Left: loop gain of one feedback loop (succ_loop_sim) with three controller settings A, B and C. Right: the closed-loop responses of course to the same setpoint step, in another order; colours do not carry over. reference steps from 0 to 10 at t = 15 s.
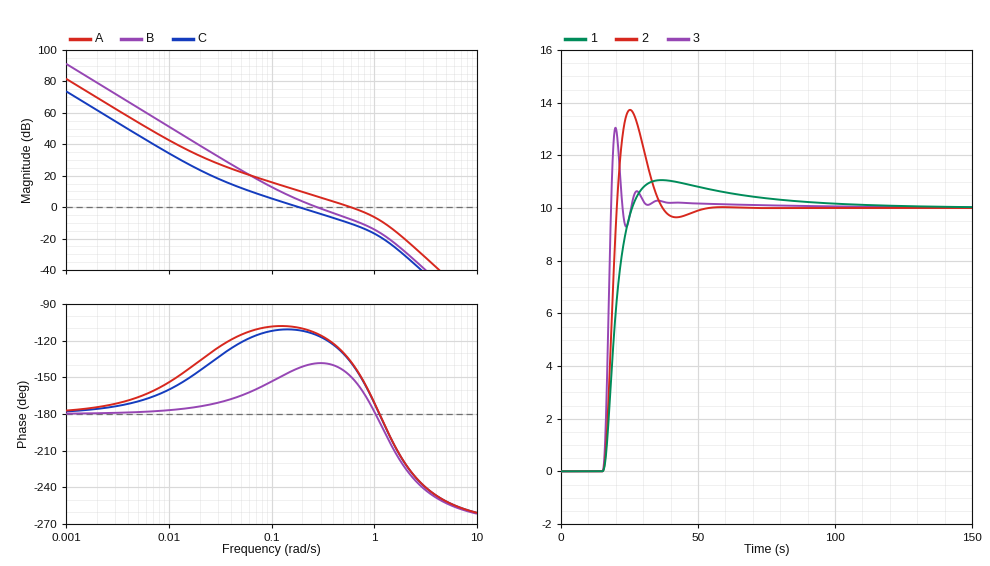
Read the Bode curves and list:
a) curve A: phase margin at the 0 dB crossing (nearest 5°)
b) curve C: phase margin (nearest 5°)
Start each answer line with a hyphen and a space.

- 45°
- 70°
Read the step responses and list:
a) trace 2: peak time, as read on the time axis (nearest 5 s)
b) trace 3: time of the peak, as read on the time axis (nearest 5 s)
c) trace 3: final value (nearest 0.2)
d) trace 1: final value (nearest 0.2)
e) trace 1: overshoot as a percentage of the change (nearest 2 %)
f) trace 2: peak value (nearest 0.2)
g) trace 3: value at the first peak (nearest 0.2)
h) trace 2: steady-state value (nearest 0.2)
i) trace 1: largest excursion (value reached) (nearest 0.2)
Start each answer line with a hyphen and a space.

- 25 s
- 20 s
- 10.0
- 10.0
- 10 %
- 13.8
- 13.0
- 10.0
- 11.0
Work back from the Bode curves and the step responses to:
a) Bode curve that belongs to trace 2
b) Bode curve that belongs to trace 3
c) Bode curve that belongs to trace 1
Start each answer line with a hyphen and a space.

- B
- A
- C
